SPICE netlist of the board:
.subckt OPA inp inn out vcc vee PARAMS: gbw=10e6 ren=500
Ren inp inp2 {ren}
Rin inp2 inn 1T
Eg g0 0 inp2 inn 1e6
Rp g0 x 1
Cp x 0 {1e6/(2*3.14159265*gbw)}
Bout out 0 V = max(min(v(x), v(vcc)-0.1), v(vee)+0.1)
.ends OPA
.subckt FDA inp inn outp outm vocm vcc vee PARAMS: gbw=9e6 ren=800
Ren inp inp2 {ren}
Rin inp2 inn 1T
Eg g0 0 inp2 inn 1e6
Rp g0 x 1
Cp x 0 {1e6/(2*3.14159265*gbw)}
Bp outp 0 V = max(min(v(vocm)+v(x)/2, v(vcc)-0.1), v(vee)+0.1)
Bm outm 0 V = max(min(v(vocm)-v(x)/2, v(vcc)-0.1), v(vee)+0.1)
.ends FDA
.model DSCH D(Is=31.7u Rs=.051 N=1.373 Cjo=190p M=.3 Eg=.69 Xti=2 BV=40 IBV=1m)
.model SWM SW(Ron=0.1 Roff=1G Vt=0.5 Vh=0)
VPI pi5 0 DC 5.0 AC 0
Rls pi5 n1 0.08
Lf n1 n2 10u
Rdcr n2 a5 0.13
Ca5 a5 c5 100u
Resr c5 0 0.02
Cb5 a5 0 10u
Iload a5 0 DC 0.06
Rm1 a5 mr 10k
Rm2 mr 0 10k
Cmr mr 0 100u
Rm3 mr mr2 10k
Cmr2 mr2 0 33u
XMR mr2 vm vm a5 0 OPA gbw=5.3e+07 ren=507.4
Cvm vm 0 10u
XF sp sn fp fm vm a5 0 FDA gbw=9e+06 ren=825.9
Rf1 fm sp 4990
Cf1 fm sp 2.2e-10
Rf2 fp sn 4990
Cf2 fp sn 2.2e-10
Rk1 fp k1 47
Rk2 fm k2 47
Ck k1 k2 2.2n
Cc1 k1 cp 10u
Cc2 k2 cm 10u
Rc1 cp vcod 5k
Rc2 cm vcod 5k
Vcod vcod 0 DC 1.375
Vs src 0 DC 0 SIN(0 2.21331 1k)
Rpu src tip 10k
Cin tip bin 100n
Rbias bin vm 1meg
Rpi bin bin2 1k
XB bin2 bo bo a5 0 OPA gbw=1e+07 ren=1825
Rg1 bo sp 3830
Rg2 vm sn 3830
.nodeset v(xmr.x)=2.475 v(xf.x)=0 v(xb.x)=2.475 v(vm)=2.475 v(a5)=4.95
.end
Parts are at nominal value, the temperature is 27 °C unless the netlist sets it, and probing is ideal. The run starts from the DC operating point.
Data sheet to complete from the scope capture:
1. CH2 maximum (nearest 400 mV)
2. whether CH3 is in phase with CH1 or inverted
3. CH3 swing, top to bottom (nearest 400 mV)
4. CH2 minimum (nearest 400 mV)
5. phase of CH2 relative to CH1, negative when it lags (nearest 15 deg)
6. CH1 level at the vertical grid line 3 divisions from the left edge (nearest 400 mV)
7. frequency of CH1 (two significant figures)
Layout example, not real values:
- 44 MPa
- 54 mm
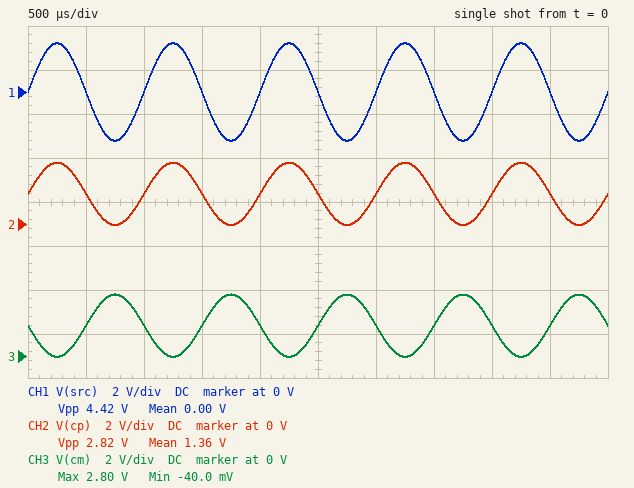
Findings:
- 2.8 V
- inverted
- 2.8 V
- 0 V
- 0 deg
- 0 V
- 1.0 kHz
